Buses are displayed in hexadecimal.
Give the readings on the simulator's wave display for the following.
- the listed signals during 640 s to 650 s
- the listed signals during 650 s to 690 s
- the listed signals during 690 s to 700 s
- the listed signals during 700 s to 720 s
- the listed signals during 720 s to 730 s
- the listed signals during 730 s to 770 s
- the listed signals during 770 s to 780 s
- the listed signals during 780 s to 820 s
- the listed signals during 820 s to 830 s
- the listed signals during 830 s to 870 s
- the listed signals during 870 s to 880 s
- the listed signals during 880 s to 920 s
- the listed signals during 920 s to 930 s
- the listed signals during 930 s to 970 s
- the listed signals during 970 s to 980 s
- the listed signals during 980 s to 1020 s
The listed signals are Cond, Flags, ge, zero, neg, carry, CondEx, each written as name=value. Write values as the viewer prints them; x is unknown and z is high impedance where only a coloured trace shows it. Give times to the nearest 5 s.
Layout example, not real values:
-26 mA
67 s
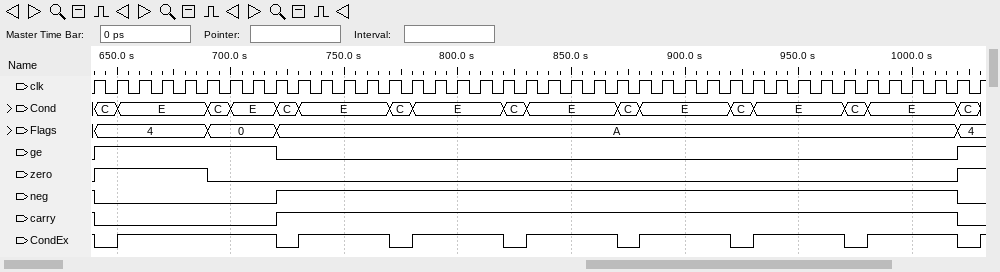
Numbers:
Cond=C, Flags=4, ge=1, zero=1, neg=0, carry=0, CondEx=0
Cond=E, Flags=4, ge=1, zero=1, neg=0, carry=0, CondEx=1
Cond=C, Flags=0, ge=1, zero=0, neg=0, carry=0, CondEx=1
Cond=E, Flags=0, ge=1, zero=0, neg=0, carry=0, CondEx=1
Cond=C, Flags=A, ge=0, zero=0, neg=1, carry=1, CondEx=0
Cond=E, Flags=A, ge=0, zero=0, neg=1, carry=1, CondEx=1
Cond=C, Flags=A, ge=0, zero=0, neg=1, carry=1, CondEx=0
Cond=E, Flags=A, ge=0, zero=0, neg=1, carry=1, CondEx=1
Cond=C, Flags=A, ge=0, zero=0, neg=1, carry=1, CondEx=0
Cond=E, Flags=A, ge=0, zero=0, neg=1, carry=1, CondEx=1
Cond=C, Flags=A, ge=0, zero=0, neg=1, carry=1, CondEx=0
Cond=E, Flags=A, ge=0, zero=0, neg=1, carry=1, CondEx=1
Cond=C, Flags=A, ge=0, zero=0, neg=1, carry=1, CondEx=0
Cond=E, Flags=A, ge=0, zero=0, neg=1, carry=1, CondEx=1
Cond=C, Flags=A, ge=0, zero=0, neg=1, carry=1, CondEx=0
Cond=E, Flags=A, ge=0, zero=0, neg=1, carry=1, CondEx=1
